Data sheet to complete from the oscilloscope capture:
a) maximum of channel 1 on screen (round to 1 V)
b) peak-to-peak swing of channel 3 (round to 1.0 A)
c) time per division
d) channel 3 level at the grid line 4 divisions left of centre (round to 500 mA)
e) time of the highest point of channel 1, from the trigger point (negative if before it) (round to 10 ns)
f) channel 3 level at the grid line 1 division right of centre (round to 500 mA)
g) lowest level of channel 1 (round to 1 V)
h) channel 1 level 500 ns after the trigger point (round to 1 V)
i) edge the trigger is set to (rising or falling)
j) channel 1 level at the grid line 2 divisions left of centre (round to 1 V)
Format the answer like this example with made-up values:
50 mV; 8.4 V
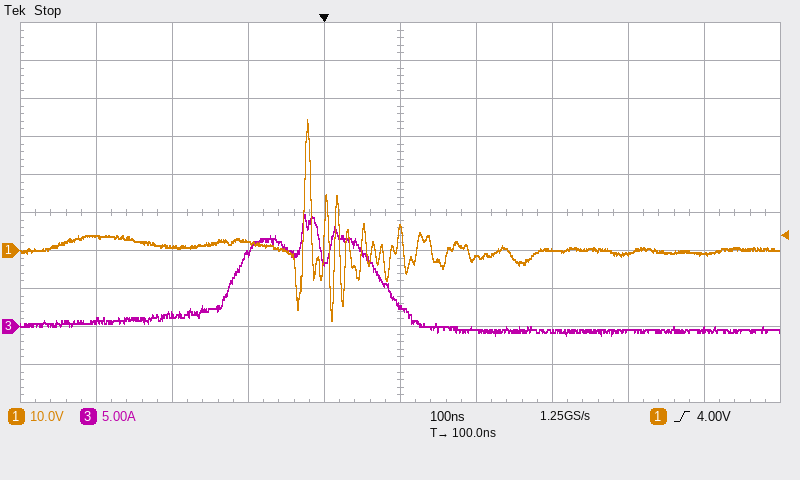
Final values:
34 V; 16.0 A; 100 ns; 1.0 A; -20 ns; -500 mA; -18 V; -1 V; rising; 2 V
